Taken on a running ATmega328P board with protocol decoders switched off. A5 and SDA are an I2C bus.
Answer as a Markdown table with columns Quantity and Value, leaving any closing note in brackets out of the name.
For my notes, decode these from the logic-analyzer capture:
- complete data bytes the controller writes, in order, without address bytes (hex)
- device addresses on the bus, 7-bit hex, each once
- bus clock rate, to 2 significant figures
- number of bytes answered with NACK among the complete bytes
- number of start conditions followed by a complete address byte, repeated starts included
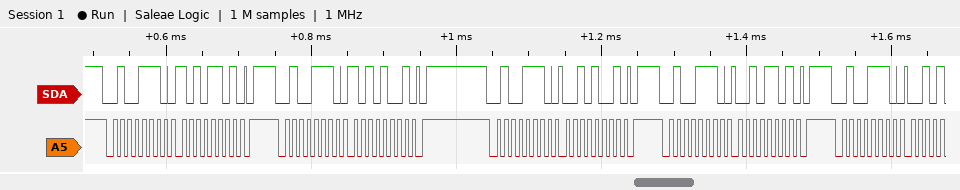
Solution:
| Quantity | Value |
|---|---|
| complete data bytes the controller writes, in order, without address bytes | AD A9 29 2D |
| device addresses on the bus, 7-bit hex, each once | 0x27 |
| bus clock rate, to 2 significant figures | 100 kHz |
| number of bytes answered with NACK among the complete bytes | 0 |
| number of start conditions followed by a complete address byte, repeated starts included | 5 |
